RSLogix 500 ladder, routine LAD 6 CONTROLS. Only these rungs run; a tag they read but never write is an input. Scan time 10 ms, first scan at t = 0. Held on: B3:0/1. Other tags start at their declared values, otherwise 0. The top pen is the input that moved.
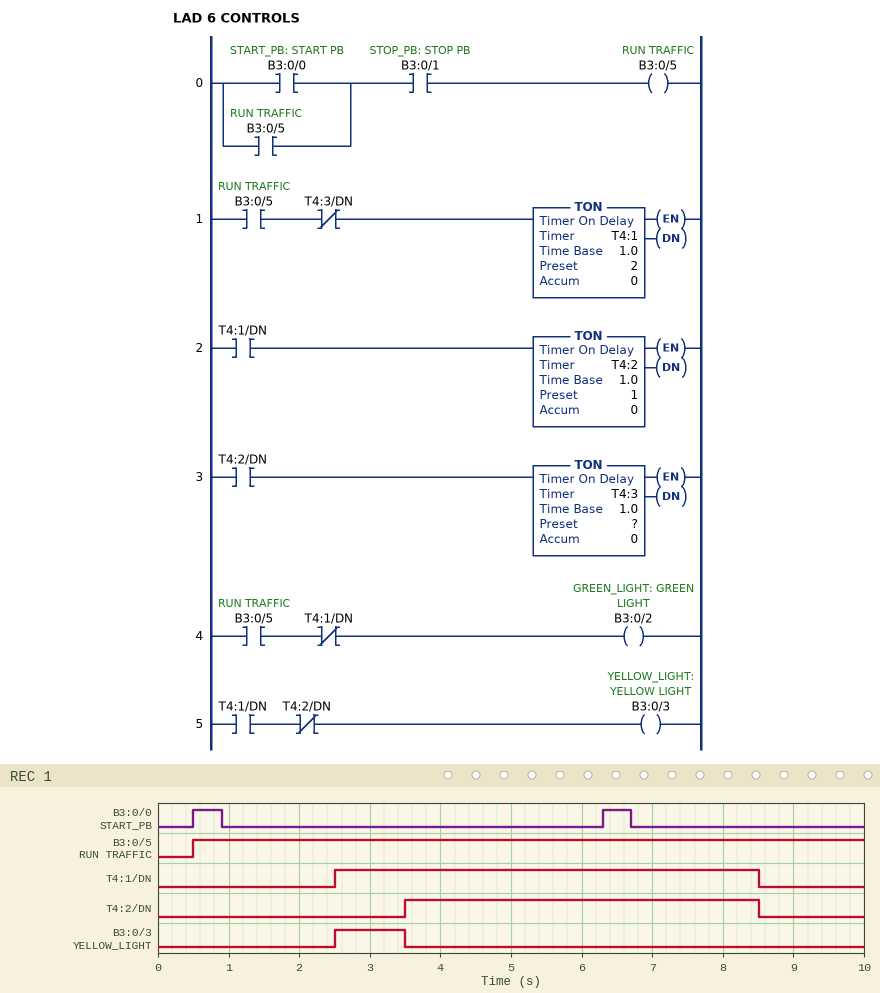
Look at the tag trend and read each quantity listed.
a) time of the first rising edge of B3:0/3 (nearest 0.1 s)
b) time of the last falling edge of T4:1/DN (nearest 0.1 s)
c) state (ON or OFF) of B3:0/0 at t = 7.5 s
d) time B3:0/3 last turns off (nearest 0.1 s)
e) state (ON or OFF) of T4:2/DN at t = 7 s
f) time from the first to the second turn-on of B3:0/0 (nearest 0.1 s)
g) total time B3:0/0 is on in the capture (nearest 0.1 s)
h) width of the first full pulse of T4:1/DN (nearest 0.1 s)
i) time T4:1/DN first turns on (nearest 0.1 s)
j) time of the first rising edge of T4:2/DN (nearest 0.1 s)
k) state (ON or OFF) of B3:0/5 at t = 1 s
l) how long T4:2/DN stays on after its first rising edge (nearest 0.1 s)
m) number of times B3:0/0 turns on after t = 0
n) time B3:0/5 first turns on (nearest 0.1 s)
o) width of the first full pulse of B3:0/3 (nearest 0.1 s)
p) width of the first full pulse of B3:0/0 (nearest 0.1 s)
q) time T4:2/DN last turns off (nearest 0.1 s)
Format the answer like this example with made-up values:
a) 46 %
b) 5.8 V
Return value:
a) 2.5 s
b) 8.5 s
c) OFF
d) 3.5 s
e) ON
f) 5.8 s
g) 0.8 s
h) 6.0 s
i) 2.5 s
j) 3.5 s
k) ON
l) 5.0 s
m) 2
n) 0.5 s
o) 1.0 s
p) 0.4 s
q) 8.5 s
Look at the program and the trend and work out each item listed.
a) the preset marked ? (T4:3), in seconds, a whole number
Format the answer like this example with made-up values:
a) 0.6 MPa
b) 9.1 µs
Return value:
a) 5 s
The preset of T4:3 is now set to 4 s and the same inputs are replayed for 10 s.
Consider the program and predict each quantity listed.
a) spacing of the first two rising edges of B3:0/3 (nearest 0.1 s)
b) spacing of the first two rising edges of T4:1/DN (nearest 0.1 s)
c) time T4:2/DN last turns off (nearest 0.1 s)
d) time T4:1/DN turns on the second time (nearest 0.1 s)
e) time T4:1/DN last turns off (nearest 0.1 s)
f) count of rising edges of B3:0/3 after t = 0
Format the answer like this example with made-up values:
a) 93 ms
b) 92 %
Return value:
a) 7.0 s
b) 7.0 s
c) 7.5 s
d) 9.5 s
e) 7.5 s
f) 2
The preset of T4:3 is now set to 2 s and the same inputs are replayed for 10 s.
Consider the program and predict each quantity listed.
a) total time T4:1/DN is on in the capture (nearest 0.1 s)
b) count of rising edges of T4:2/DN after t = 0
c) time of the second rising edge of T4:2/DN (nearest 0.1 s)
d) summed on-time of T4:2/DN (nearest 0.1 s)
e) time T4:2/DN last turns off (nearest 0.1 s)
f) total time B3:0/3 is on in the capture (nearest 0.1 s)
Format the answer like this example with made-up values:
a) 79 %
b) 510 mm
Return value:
a) 5.5 s
b) 2
c) 8.5 s
d) 3.5 s
e) 5.5 s
f) 2.0 s
